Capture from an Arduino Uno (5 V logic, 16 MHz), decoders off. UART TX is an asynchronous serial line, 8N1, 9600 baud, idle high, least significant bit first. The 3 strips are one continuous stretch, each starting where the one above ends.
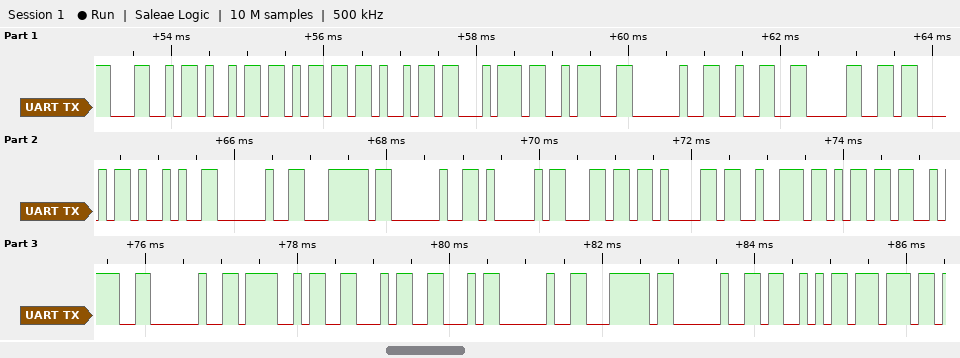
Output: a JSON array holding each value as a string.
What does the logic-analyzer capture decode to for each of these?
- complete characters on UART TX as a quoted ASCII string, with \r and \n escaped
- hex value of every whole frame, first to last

["\"Limit: 20C) | Alarm: OFF | Sw\"", "4C 69 6D 69 74 3A 20 32 30 43 29 20 7C 20 41 6C 61 72 6D 3A 20 4F 46 46 20 7C 20 53 77"]
